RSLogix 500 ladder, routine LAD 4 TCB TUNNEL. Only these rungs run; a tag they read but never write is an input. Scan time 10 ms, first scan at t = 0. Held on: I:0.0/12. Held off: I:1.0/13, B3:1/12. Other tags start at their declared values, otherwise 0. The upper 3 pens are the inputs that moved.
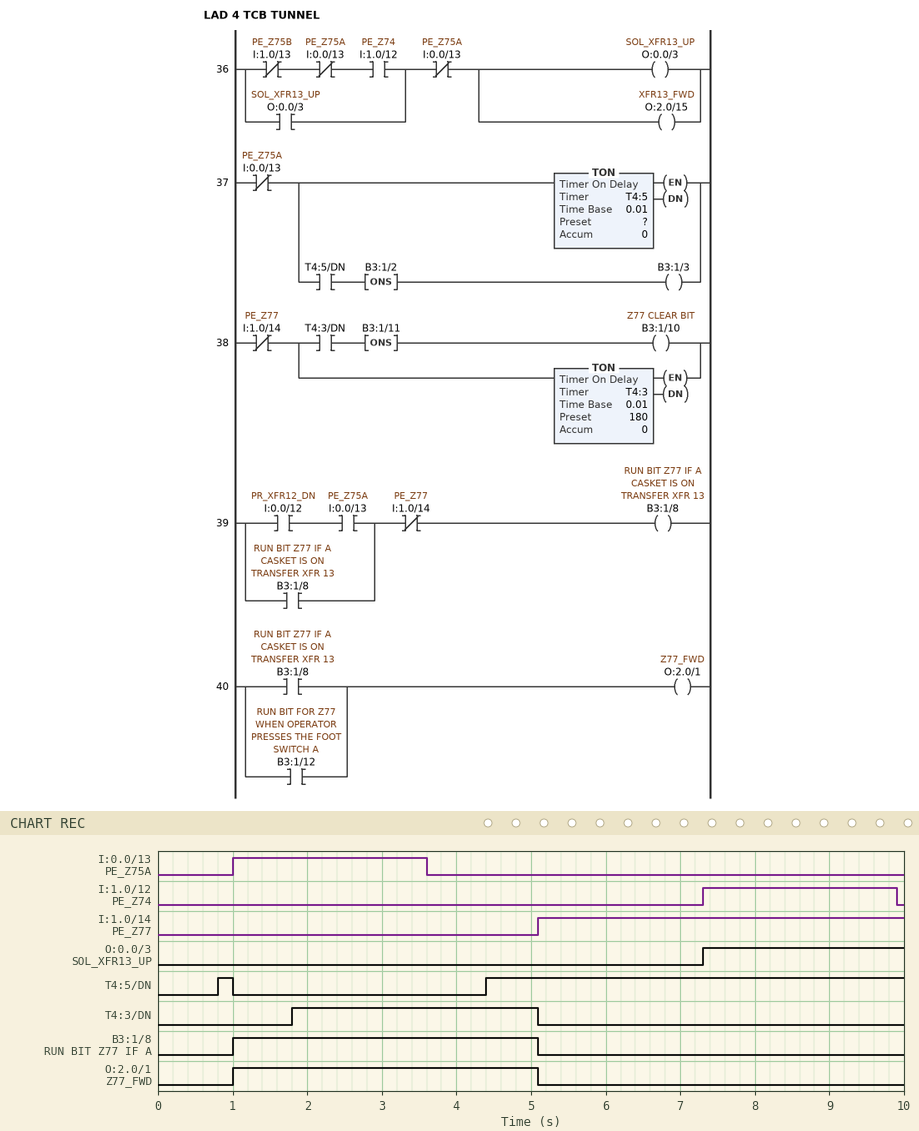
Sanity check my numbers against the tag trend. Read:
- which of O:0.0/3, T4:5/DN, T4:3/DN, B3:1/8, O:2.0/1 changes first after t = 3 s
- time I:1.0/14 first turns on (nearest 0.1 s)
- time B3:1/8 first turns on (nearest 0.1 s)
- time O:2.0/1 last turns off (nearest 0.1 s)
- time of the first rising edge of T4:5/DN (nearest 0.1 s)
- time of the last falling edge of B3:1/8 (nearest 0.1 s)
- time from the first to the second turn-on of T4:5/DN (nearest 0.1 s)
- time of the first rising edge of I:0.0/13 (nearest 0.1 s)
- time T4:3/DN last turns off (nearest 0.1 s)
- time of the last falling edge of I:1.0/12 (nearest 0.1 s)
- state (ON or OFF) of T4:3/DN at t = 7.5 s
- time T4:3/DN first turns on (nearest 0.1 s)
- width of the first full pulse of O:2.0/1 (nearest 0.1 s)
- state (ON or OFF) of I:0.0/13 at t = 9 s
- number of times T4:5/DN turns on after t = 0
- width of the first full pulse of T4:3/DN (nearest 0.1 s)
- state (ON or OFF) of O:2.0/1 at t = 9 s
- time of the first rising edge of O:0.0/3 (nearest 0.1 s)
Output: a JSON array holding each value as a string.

["T4:5/DN", "5.1 s", "1.0 s", "5.1 s", "0.8 s", "5.1 s", "3.6 s", "1.0 s", "5.1 s", "9.9 s", "OFF", "1.8 s", "4.1 s", "OFF", "2", "3.3 s", "OFF", "7.3 s"]
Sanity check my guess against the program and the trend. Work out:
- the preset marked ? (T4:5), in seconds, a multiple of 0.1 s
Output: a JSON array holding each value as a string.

["0.8 s"]
